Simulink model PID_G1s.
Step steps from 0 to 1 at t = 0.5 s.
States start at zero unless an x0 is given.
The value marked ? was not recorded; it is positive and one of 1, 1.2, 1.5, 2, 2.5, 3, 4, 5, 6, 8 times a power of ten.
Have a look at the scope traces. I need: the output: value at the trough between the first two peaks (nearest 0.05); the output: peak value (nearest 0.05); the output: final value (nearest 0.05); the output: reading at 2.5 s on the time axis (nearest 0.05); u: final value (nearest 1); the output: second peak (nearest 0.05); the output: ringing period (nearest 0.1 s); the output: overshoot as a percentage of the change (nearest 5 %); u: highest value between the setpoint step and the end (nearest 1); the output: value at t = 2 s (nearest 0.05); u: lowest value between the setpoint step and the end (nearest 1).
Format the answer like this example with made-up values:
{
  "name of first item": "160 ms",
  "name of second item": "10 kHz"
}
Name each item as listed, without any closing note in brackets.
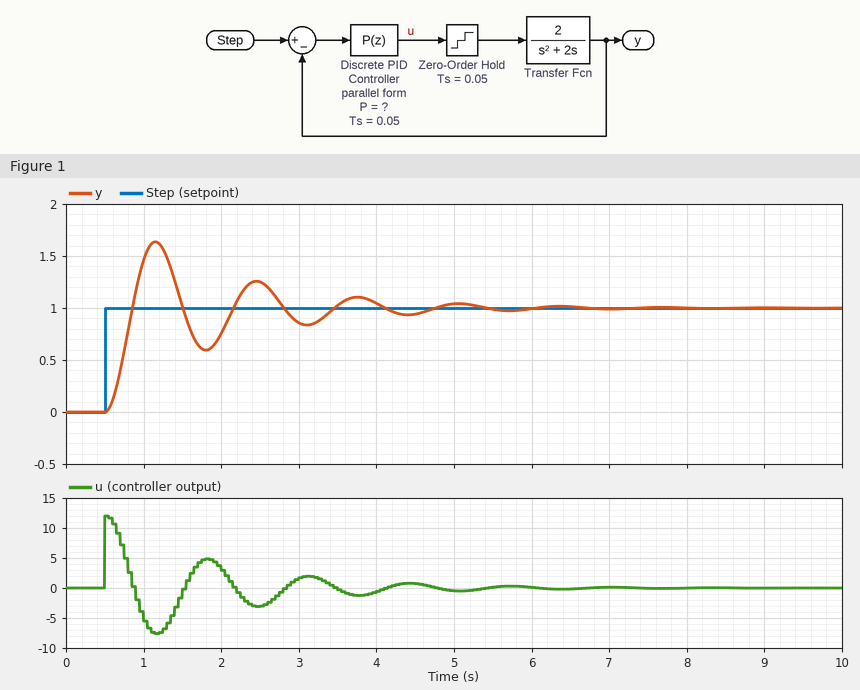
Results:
{
  "the output: value at the trough between the first two peaks": "0.60",
  "the output: peak value": "1.65",
  "the output: final value": "1.00",
  "the output: reading at 2.5 s on the time axis": "1.25",
  "u: final value": "0",
  "the output: second peak": "1.25",
  "the output: ringing period": "1.3 s",
  "the output: overshoot as a percentage of the change": "65 %",
  "u: highest value between the setpoint step and the end": "12",
  "the output: value at t = 2 s": "0.75",
  "u: lowest value between the setpoint step and the end": "-8"
}
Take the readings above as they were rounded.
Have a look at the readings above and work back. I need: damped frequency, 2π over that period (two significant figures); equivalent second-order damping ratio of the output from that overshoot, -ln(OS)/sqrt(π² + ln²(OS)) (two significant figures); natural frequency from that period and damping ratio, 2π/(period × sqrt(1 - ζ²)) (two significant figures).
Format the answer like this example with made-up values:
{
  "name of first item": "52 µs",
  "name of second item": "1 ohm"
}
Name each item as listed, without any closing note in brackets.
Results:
{
  "damped frequency, 2π over that period": "4.8 rad/s",
  "equivalent second-order damping ratio of the output from that overshoot, -ln(OS)/sqrt(π² + ln²(OS))": "0.14",
  "natural frequency from that period and damping ratio, 2π/(period × sqrt(1 - ζ²))": "4.9 rad/s"
}
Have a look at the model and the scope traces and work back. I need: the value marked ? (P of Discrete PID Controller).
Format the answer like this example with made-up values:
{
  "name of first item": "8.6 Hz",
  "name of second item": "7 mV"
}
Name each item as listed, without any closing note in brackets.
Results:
{
  "the value marked ?": "12"
}
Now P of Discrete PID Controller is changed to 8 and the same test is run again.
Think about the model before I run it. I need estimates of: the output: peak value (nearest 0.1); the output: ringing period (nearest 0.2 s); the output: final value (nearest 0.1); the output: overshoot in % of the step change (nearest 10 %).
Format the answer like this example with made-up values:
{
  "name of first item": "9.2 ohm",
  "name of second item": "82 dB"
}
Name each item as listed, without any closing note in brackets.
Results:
{
  "the output: peak value": "1.5",
  "the output: ringing period": "1.6 s",
  "the output: final value": "1.0",
  "the output: overshoot in % of the step change": "50 %"
}
